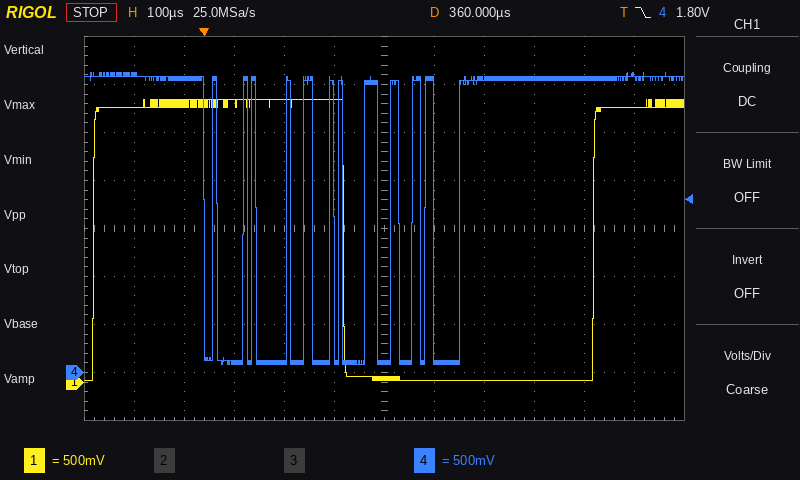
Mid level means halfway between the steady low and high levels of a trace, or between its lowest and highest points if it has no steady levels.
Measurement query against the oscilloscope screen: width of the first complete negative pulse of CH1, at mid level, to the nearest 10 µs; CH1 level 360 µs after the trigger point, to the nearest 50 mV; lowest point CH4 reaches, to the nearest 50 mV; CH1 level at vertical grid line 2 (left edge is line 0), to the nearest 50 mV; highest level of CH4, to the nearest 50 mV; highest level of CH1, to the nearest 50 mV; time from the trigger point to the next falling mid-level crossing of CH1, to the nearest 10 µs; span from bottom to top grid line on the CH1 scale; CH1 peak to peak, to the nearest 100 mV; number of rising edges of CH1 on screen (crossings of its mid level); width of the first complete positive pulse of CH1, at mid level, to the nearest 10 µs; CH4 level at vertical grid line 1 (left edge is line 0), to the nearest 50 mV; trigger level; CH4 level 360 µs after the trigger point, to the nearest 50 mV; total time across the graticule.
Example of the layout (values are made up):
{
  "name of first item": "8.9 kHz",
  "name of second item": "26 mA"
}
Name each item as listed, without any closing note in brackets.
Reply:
{
  "width of the first complete negative pulse of CH1, at mid level, to the nearest 10 µs": "500 µs",
  "CH1 level 360 µs after the trigger point, to the nearest 50 mV": "50 mV",
  "lowest point CH4 reaches, to the nearest 50 mV": "100 mV",
  "CH1 level at vertical grid line 2 (left edge is line 0), to the nearest 50 mV": "2.90 V",
  "highest level of CH4, to the nearest 50 mV": "3.10 V",
  "highest level of CH1, to the nearest 50 mV": "2.95 V",
  "time from the trigger point to the next falling mid-level crossing of CH1, to the nearest 10 µs": "280 µs",
  "span from bottom to top grid line on the CH1 scale": "4 V",
  "CH1 peak to peak, to the nearest 100 mV": "2.90 V",
  "number of rising edges of CH1 on screen": "2",
  "width of the first complete positive pulse of CH1, at mid level, to the nearest 10 µs": "500 µs",
  "CH4 level at vertical grid line 1 (left edge is line 0), to the nearest 50 mV": "3.10 V",
  "trigger level": "1.80 V",
  "CH4 level 360 µs after the trigger point, to the nearest 50 mV": "100 mV",
  "total time across the graticule": "1.2 ms"
}
